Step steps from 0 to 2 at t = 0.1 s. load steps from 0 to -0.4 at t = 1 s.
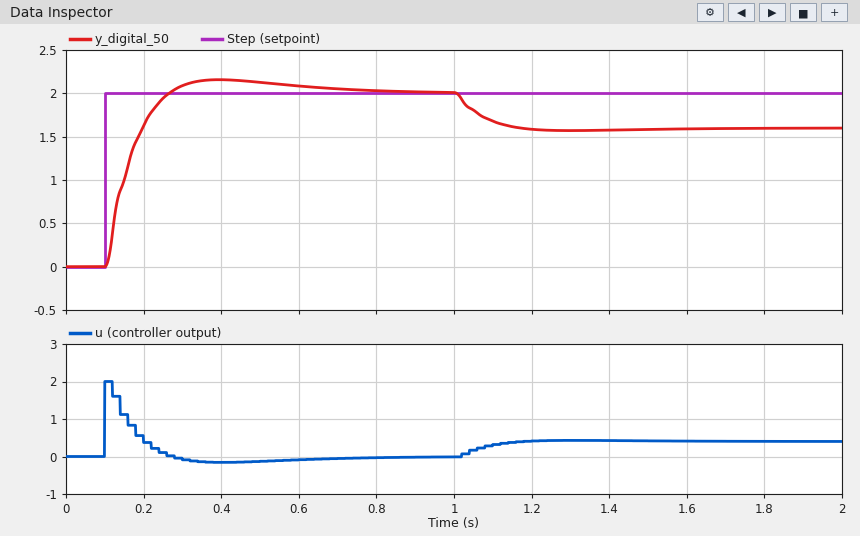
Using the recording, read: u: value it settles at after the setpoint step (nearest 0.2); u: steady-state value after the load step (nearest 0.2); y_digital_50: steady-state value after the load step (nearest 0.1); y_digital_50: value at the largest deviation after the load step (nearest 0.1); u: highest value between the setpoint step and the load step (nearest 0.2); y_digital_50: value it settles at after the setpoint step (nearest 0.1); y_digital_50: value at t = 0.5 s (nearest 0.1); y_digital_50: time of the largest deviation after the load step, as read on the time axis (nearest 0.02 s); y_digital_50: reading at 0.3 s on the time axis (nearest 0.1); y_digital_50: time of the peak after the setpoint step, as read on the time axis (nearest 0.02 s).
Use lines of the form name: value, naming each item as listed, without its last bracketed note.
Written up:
u: value it settles at after the setpoint step: 0.0
u: steady-state value after the load step: 0.4
y_digital_50: steady-state value after the load step: 1.6
y_digital_50: value at the largest deviation after the load step: 1.6
u: highest value between the setpoint step and the load step: 2.0
y_digital_50: value it settles at after the setpoint step: 2.0
y_digital_50: value at t = 0.5 s: 2.1
y_digital_50: time of the largest deviation after the load step, as read on the time axis: 1.30 s
y_digital_50: reading at 0.3 s on the time axis: 2.1
y_digital_50: time of the peak after the setpoint step, as read on the time axis: 0.40 s
